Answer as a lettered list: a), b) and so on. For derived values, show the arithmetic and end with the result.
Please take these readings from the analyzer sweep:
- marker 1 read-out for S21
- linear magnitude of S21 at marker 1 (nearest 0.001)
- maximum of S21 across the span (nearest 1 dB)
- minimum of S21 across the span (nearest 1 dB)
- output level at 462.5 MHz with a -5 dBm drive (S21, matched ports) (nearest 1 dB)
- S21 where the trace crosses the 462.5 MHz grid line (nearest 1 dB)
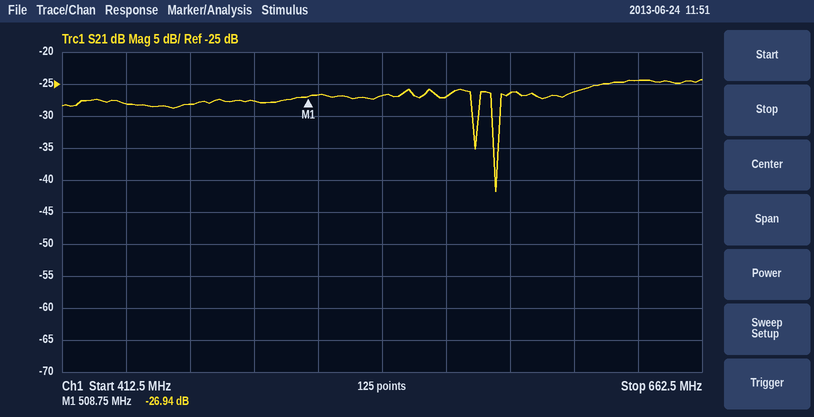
a) -26.94 dB
b) 10^(-26.94/20) ≈ 0.045
c) -24 dB
d) -42 dB
e) -5 dBm + (-28 dB) = -33 dBm
f) -28 dB
